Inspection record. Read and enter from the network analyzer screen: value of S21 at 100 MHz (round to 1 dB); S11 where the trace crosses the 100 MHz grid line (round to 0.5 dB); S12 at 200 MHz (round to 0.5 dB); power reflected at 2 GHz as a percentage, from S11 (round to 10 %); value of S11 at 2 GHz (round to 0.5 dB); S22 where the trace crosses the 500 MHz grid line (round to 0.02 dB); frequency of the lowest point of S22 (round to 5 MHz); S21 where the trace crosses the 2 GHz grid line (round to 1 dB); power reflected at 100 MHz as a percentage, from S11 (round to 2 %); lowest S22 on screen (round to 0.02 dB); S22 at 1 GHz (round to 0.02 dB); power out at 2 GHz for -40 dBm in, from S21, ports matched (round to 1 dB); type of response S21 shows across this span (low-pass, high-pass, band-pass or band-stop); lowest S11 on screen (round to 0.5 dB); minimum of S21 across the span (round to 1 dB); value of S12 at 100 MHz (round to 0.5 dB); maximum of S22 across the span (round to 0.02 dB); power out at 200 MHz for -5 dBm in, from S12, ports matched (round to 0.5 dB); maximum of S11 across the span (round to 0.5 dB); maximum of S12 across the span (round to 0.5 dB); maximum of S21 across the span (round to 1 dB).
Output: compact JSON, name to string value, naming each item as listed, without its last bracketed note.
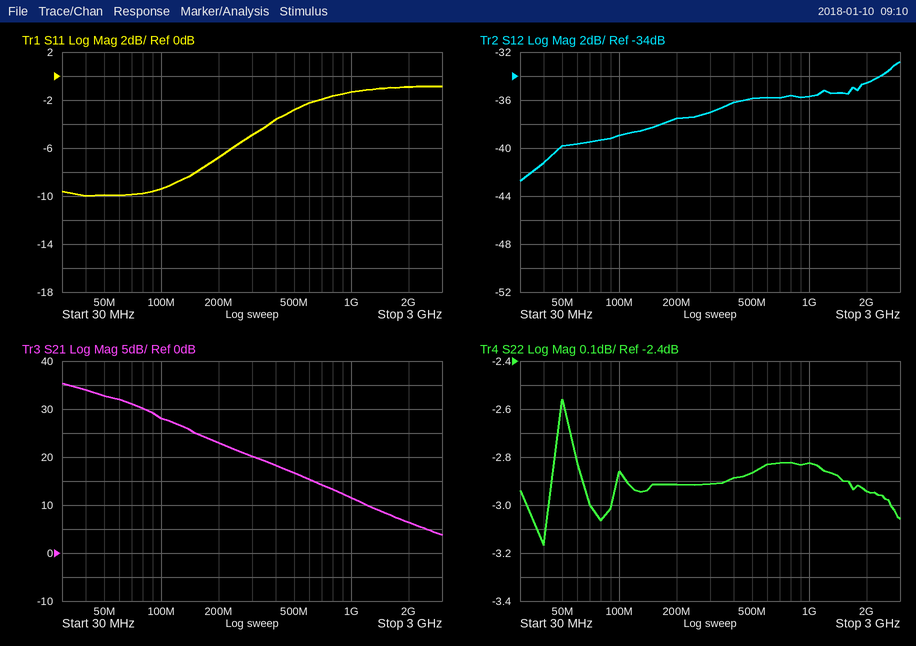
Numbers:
{"value of S21 at 100 MHz": "28 dB", "S11 where the trace crosses the 100 MHz grid line": "-9.5 dB", "S12 at 200 MHz": "-37.5 dB", "power reflected at 2 GHz as a percentage, from S11": "80 %", "value of S11 at 2 GHz": "-1.0 dB", "S22 where the trace crosses the 500 MHz grid line": "-2.86 dB", "frequency of the lowest point of S22": "40 MHz", "S21 where the trace crosses the 2 GHz grid line": "6 dB", "power reflected at 100 MHz as a percentage, from S11": "12 %", "lowest S22 on screen": "-3.16 dB", "S22 at 1 GHz": "-2.82 dB", "power out at 2 GHz for -40 dBm in, from S21, ports matched": "-34 dBm", "type of response S21 shows across this span": "low-pass", "lowest S11 on screen": "-10.0 dB", "minimum of S21 across the span": "4 dB", "value of S12 at 100 MHz": "-39.0 dB", "maximum of S22 across the span": "-2.56 dB", "power out at 200 MHz for -5 dBm in, from S12, ports matched": "-42.5 dBm", "maximum of S11 across the span": "-1.0 dB", "maximum of S12 across the span": "-33.0 dB", "maximum of S21 across the span": "35 dB"}
